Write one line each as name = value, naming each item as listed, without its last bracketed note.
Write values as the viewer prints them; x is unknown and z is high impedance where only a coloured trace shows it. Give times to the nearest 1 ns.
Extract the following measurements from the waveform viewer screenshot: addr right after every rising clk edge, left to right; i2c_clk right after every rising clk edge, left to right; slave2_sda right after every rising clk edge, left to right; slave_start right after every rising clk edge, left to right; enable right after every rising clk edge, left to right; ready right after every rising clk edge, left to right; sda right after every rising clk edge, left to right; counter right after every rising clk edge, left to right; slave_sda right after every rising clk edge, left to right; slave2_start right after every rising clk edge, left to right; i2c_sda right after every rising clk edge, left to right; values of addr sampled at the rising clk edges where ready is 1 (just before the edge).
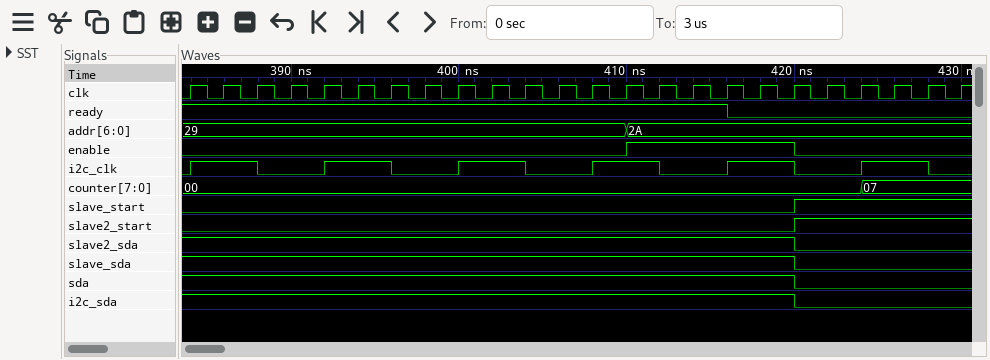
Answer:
addr right after every rising clk edge, left to right = 29, 29, 29, 29, 29, 29, 29, 29, 29, 29, 29, 29, 29, 2A, 2A, 2A, 2A, 2A, 2A, 2A, 2A, 2A, 2A, 2A
i2c_clk right after every rising clk edge, left to right = 1 1 0 0 1 1 0 0 1 1 0 0 1 1 0 0 1 1 0 0 1 1 0 0
slave2_sda right after every rising clk edge, left to right = 1 1 1 1 1 1 1 1 1 1 1 1 1 1 1 1 1 1 0 0 0 0 0 0
slave_start right after every rising clk edge, left to right = 0 0 0 0 0 0 0 0 0 0 0 0 0 0 0 0 0 0 1 1 1 1 1 1
enable right after every rising clk edge, left to right = 0 0 0 0 0 0 0 0 0 0 0 0 0 1 1 1 1 1 0 0 0 0 0 0
ready right after every rising clk edge, left to right = 1 1 1 1 1 1 1 1 1 1 1 1 1 1 1 1 0 0 0 0 0 0 0 0
sda right after every rising clk edge, left to right = 1 1 1 1 1 1 1 1 1 1 1 1 1 1 1 1 1 1 0 0 0 0 0 0
counter right after every rising clk edge, left to right = 00, 00, 00, 00, 00, 00, 00, 00, 00, 00, 00, 00, 00, 00, 00, 00, 00, 00, 00, 00, 07, 07, 07, 07
slave_sda right after every rising clk edge, left to right = 1 1 1 1 1 1 1 1 1 1 1 1 1 1 1 1 1 1 0 0 0 0 0 0
slave2_start right after every rising clk edge, left to right = 0 0 0 0 0 0 0 0 0 0 0 0 0 0 0 0 0 0 1 1 1 1 1 1
i2c_sda right after every rising clk edge, left to right = 1 1 1 1 1 1 1 1 1 1 1 1 1 1 1 1 1 1 0 0 0 0 0 0
values of addr sampled at the rising clk edges where ready is 1 = 29, 29, 29, 29, 29, 29, 29, 29, 29, 29, 29, 29, 29, 29, 2A, 2A, 2A
